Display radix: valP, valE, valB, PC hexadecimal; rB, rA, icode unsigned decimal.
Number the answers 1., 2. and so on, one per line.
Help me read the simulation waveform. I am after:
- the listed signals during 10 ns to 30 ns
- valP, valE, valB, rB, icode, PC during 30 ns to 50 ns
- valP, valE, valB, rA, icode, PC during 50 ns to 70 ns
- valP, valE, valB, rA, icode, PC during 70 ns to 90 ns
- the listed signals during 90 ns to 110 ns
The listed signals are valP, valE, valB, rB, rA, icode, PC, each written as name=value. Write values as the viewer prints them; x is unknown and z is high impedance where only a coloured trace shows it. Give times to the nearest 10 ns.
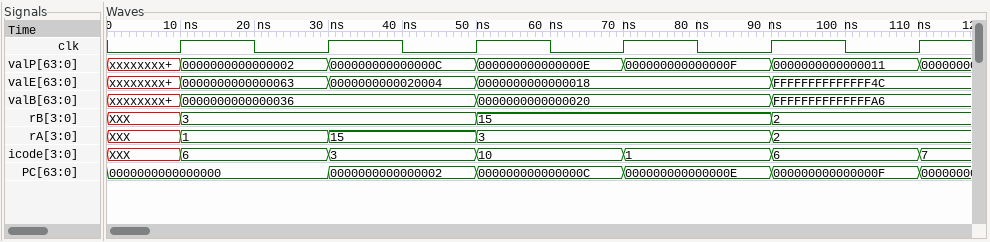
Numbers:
1. valP=0000000000000002, valE=0000000000000063, valB=0000000000000036, rB=3, rA=1, icode=6, PC=0000000000000000
2. valP=000000000000000C, valE=0000000000020004, valB=0000000000000036, rB=3, icode=3, PC=0000000000000002
3. valP=000000000000000E, valE=0000000000000018, valB=0000000000000020, rA=3, icode=10, PC=000000000000000C
4. valP=000000000000000F, valE=0000000000000018, valB=0000000000000020, rA=3, icode=1, PC=000000000000000E
5. valP=0000000000000011, valE=FFFFFFFFFFFFFF4C, valB=FFFFFFFFFFFFFFA6, rB=2, rA=2, icode=6, PC=000000000000000F
